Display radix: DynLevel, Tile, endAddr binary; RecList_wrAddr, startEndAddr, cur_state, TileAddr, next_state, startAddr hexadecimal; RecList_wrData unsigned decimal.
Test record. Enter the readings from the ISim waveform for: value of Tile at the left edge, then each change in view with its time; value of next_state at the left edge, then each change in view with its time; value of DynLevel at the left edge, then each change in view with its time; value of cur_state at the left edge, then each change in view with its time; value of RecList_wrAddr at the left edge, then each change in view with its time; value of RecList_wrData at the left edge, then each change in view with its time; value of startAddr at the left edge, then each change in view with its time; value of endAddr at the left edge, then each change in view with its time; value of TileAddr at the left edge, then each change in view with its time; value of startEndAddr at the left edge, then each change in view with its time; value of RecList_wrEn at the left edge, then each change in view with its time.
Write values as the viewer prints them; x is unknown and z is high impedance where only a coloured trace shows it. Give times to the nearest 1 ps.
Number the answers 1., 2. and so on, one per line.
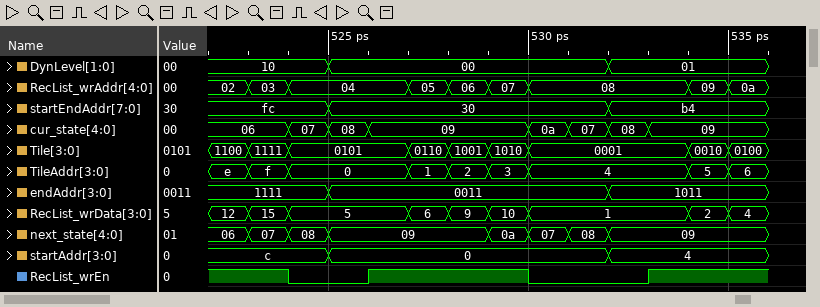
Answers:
1. 1100, 1111 at 523 ps, 0101 at 524 ps, 0110 at 527 ps, 1001 at 528 ps, 1010 at 529 ps, 0001 at 530 ps, 0010 at 534 ps, 0100 at 535 ps
2. 06, 07 at 523 ps, 08 at 524 ps, 09 at 525 ps, 0a at 529 ps, 07 at 530 ps, 08 at 531 ps, 09 at 532 ps
3. 10, 00 at 525 ps, 01 at 532 ps
4. 06, 07 at 524 ps, 08 at 525 ps, 09 at 526 ps, 0a at 530 ps, 07 at 531 ps, 08 at 532 ps, 09 at 533 ps
5. 02, 03 at 523 ps, 04 at 524 ps, 05 at 527 ps, 06 at 528 ps, 07 at 529 ps, 08 at 530 ps, 09 at 534 ps, 0a at 535 ps
6. 12, 15 at 523 ps, 5 at 524 ps, 6 at 527 ps, 9 at 528 ps, 10 at 529 ps, 1 at 530 ps, 2 at 534 ps, 4 at 535 ps
7. c, 0 at 525 ps, 4 at 532 ps
8. 1111, 0011 at 525 ps, 1011 at 532 ps
9. e, f at 523 ps, 0 at 524 ps, 1 at 527 ps, 2 at 528 ps, 3 at 529 ps, 4 at 530 ps, 5 at 534 ps, 6 at 535 ps
10. fc, 30 at 525 ps, b4 at 532 ps
11. 1, 0 at 524 ps, 1 at 526 ps, 0 at 530 ps, 1 at 533 ps
